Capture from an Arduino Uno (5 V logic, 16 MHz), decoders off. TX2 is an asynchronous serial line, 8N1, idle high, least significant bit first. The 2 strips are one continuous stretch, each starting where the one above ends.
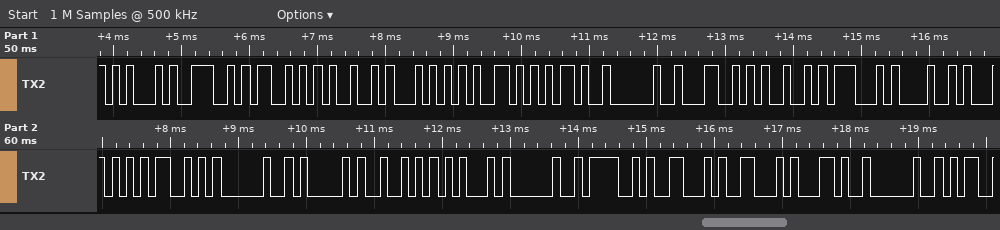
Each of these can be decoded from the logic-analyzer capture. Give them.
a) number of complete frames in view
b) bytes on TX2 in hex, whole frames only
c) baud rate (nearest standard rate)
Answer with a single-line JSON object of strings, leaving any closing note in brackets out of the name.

{"number of complete frames in view": "24", "bytes on TX2 in hex, whole frames only": "45 4E 53 49 54 59 2D 20 4C 49 47 48 54 53 20 41 52 45 20 4F 46 46 2C 20", "baud rate": "9600 baud"}
